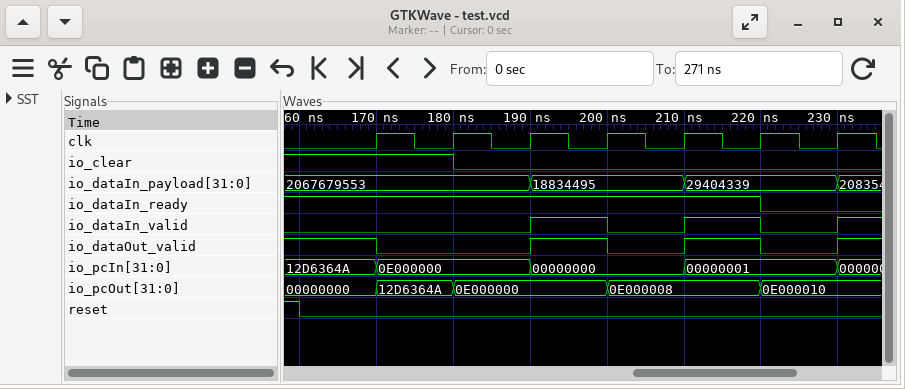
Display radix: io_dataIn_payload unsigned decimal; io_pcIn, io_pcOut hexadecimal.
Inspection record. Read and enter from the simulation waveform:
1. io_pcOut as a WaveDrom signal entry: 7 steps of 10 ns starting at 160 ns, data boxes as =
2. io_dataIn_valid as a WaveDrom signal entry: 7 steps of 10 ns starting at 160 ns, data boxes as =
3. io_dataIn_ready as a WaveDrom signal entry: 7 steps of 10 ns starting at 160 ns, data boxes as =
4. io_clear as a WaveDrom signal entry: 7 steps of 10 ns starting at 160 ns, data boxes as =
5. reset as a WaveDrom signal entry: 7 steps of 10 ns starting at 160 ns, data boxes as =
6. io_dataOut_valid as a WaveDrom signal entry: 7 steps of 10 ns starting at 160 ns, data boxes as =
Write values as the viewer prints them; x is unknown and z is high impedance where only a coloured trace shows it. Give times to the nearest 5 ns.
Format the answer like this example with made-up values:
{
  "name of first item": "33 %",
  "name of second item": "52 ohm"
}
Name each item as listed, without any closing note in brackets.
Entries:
{
  "io_pcOut as a WaveDrom signal entry: 7 steps of 10 ns starting at 160 ns, data boxes as =": "{name: 'io_pcOut', wave: '===.=.=', data: '00000000 12D6364A 0E000000 0E000008 0E000010'}",
  "io_dataIn_valid as a WaveDrom signal entry: 7 steps of 10 ns starting at 160 ns, data boxes as =": "{name: 'io_dataIn_valid', wave: '0..1010'}",
  "io_dataIn_ready as a WaveDrom signal entry: 7 steps of 10 ns starting at 160 ns, data boxes as =": "{name: 'io_dataIn_ready', wave: '1.....0'}",
  "io_clear as a WaveDrom signal entry: 7 steps of 10 ns starting at 160 ns, data boxes as =": "{name: 'io_clear', wave: '1.0....'}",
  "reset as a WaveDrom signal entry: 7 steps of 10 ns starting at 160 ns, data boxes as =": "{name: 'reset', wave: '0......'}",
  "io_dataOut_valid as a WaveDrom signal entry: 7 steps of 10 ns starting at 160 ns, data boxes as =": "{name: 'io_dataOut_valid', wave: '10.1010'}"
}
